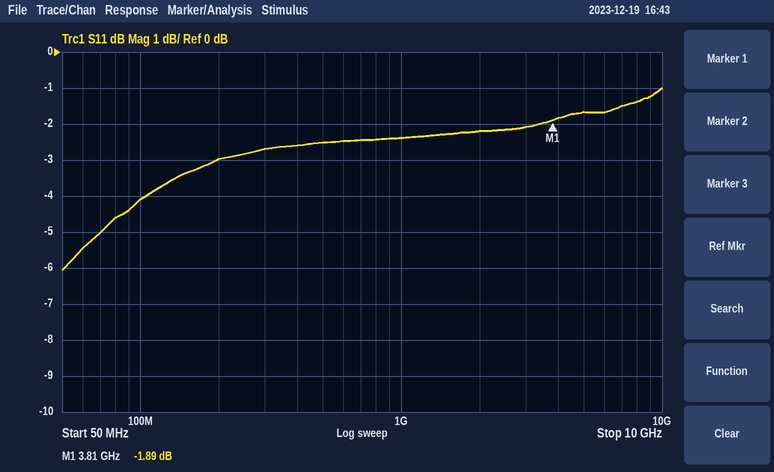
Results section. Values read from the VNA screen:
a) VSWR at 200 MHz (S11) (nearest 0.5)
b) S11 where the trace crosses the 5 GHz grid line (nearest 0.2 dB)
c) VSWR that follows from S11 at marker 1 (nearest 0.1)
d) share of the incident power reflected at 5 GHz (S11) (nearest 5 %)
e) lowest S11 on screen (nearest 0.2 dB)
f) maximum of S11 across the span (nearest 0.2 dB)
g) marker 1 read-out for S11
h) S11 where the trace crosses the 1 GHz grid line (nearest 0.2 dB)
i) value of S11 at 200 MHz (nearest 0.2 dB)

6.0
-1.6 dB
9.2
70 %
-6.0 dB
-1.0 dB
-1.89 dB
-2.4 dB
-3.0 dB
